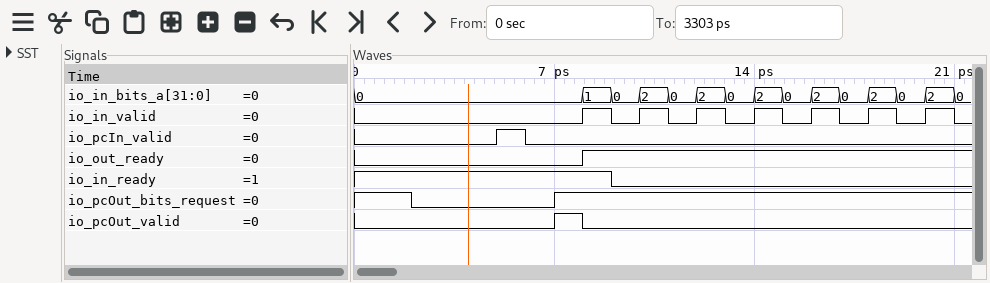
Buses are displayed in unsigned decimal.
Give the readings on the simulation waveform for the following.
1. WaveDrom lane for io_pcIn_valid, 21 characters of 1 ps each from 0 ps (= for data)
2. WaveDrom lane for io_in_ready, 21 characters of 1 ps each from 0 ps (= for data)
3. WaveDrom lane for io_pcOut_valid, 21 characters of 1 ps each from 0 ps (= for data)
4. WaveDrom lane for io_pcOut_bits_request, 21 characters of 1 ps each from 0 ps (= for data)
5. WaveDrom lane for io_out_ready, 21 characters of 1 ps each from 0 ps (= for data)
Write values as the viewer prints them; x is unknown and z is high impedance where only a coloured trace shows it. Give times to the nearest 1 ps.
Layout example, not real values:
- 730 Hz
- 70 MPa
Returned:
- {name: 'io_pcIn_valid', wave: '0....10..............'}
- {name: 'io_in_ready', wave: '1........0...........'}
- {name: 'io_pcOut_valid', wave: '0......10............'}
- {name: 'io_pcOut_bits_request', wave: '1.0....1.............'}
- {name: 'io_out_ready', wave: '0.......1............'}
